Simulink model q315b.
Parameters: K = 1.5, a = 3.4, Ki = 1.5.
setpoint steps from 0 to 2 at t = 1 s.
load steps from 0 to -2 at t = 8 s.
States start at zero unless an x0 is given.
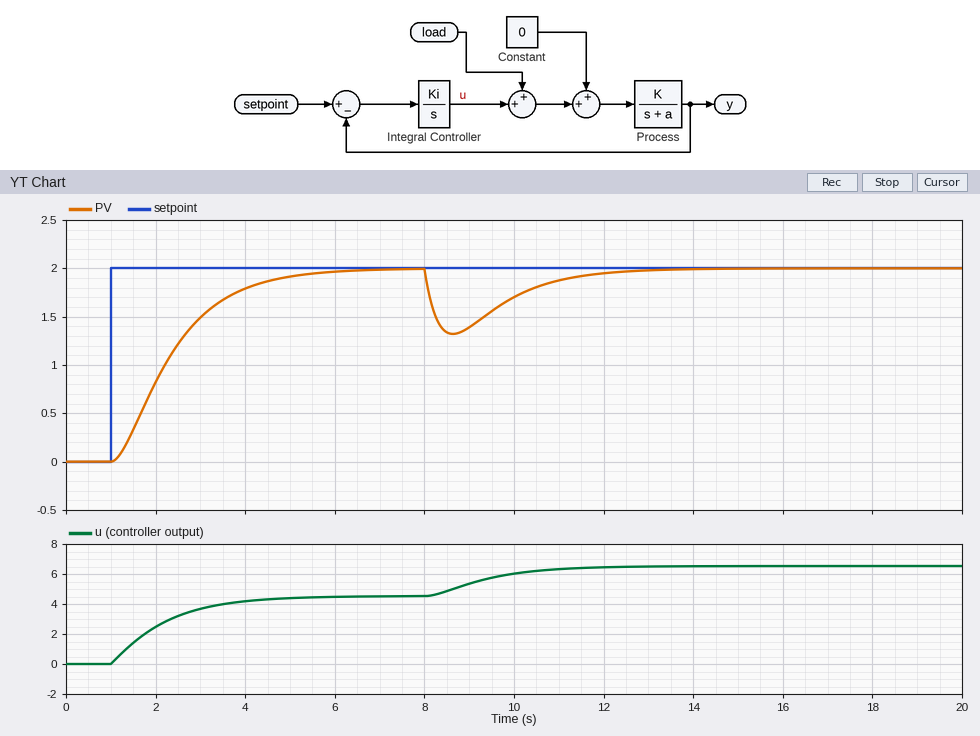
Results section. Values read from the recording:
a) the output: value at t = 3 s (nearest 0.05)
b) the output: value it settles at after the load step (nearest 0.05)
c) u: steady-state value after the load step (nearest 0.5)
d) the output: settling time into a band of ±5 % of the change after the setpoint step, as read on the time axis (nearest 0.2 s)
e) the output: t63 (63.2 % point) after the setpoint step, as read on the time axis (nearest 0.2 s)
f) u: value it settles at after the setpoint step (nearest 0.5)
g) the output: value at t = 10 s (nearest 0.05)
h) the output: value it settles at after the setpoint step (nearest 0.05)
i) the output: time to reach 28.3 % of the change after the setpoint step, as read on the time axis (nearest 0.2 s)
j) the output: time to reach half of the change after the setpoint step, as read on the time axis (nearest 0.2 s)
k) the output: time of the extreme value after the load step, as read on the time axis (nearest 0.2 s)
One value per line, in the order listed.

1.50
2.00
6.5
4.8 s
2.6 s
4.5
1.70
2.00
1.8 s
2.2 s
8.6 s
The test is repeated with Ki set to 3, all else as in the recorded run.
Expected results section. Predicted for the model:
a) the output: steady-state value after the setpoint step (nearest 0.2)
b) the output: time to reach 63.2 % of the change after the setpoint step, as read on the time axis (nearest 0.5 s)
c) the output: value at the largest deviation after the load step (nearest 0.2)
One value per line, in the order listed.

2.0
2.0 s
1.4
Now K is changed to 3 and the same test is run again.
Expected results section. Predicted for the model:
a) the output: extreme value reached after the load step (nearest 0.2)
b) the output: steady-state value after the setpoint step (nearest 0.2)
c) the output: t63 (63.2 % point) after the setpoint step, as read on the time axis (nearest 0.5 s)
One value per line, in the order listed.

0.8
2.0
2.0 s
